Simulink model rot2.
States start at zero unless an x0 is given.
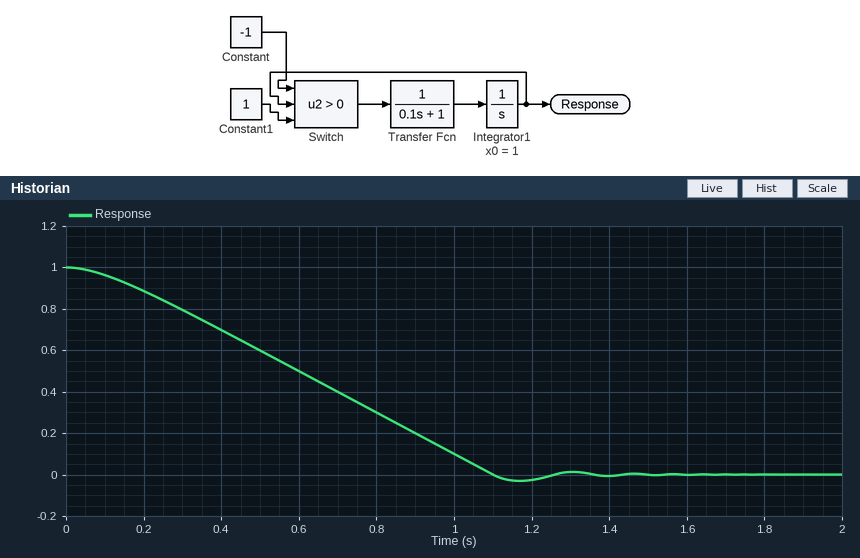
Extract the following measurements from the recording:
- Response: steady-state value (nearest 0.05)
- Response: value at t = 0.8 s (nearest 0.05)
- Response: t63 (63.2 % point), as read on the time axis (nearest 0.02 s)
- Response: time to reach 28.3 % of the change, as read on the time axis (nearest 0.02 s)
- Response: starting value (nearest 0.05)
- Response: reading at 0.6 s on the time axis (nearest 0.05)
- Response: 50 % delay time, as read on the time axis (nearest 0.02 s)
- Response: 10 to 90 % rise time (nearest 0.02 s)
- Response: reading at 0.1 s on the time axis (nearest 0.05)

0.00
0.30
0.74 s
0.38 s
1.00
0.50
0.60 s
0.82 s
0.95
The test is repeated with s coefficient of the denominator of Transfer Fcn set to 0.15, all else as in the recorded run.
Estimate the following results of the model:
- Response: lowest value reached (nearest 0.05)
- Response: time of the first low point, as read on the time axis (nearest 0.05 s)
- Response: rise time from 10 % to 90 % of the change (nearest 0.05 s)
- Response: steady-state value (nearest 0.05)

-0.05
1.25 s
0.85 s
0.00
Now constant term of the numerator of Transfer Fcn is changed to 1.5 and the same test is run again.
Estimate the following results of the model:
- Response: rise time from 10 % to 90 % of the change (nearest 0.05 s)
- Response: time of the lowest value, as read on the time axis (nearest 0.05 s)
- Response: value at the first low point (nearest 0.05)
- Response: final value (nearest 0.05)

0.55 s
0.85 s
-0.05
0.00
